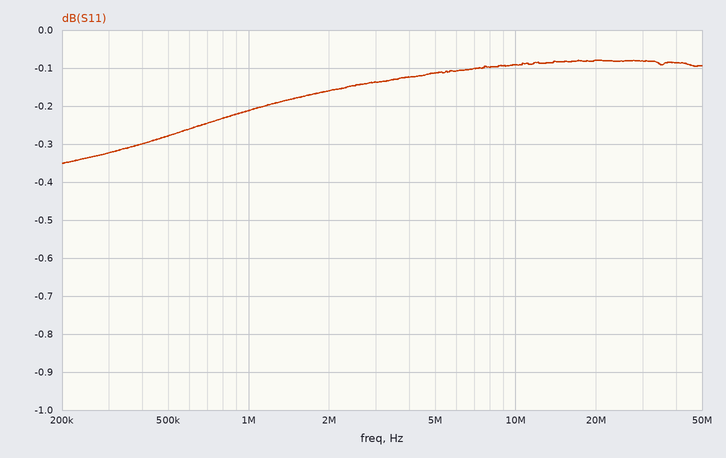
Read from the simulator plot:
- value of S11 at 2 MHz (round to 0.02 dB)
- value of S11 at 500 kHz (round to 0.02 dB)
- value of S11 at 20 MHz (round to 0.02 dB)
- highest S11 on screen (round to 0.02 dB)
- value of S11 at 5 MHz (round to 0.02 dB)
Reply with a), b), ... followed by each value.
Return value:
a) -0.16 dB
b) -0.28 dB
c) -0.08 dB
d) -0.08 dB
e) -0.12 dB
